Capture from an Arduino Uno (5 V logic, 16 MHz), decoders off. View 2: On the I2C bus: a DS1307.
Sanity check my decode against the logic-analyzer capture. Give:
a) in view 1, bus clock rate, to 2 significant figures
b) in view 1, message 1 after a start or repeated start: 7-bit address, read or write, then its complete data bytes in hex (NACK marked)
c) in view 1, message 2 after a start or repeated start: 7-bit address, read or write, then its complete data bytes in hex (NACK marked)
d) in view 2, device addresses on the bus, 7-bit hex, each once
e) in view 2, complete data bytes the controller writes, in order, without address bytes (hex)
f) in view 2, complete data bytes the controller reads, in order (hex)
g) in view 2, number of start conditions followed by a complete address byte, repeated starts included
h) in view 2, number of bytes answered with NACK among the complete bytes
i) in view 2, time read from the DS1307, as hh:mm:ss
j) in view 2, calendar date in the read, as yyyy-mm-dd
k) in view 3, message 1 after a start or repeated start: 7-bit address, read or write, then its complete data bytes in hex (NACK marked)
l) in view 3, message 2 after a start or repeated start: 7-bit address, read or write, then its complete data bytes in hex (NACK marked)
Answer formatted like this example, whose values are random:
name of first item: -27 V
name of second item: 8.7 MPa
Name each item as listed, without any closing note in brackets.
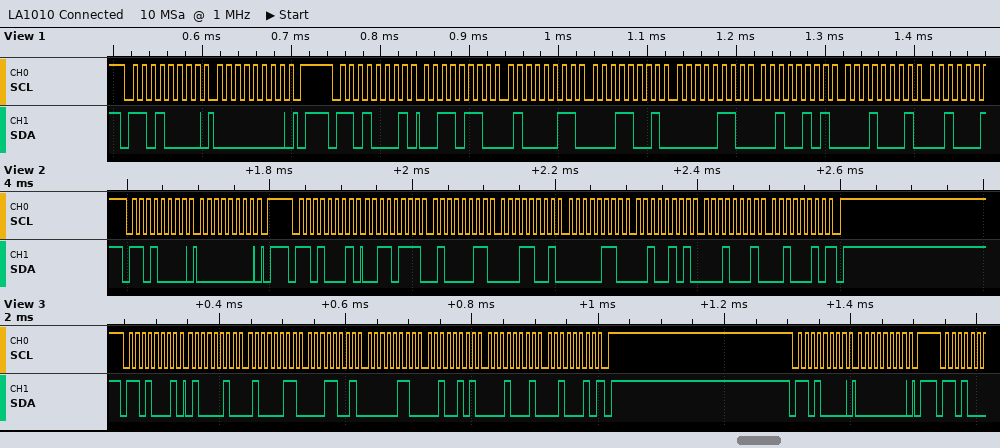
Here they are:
in view 1, bus clock rate, to 2 significant figures: 100 kHz
in view 1, message 1 after a start or repeated start: 7-bit address, read or write, then its complete data bytes in hex: 0x68 write: 00
in view 1, message 2 after a start or repeated start: 7-bit address, read or write, then its complete data bytes in hex: 0x68 read: 36 43 19 06 25 11
in view 2, device addresses on the bus, 7-bit hex, each once: 0x68
in view 2, complete data bytes the controller writes, in order, without address bytes: 00
in view 2, complete data bytes the controller reads, in order: 37 43 19 06 25 11 22
in view 2, number of start conditions followed by a complete address byte, repeated starts included: 2
in view 2, number of bytes answered with NACK among the complete bytes: 1
in view 2, time read from the DS1307, as hh:mm:ss: 19:43:37
in view 2, calendar date in the read, as yyyy-mm-dd: 2022-11-25
in view 3, message 1 after a start or repeated start: 7-bit address, read or write, then its complete data bytes in hex: 0x68 read: 42 43 19 06 25 11 22 NACK
in view 3, message 2 after a start or repeated start: 7-bit address, read or write, then its complete data bytes in hex: 0x68 write: 00
